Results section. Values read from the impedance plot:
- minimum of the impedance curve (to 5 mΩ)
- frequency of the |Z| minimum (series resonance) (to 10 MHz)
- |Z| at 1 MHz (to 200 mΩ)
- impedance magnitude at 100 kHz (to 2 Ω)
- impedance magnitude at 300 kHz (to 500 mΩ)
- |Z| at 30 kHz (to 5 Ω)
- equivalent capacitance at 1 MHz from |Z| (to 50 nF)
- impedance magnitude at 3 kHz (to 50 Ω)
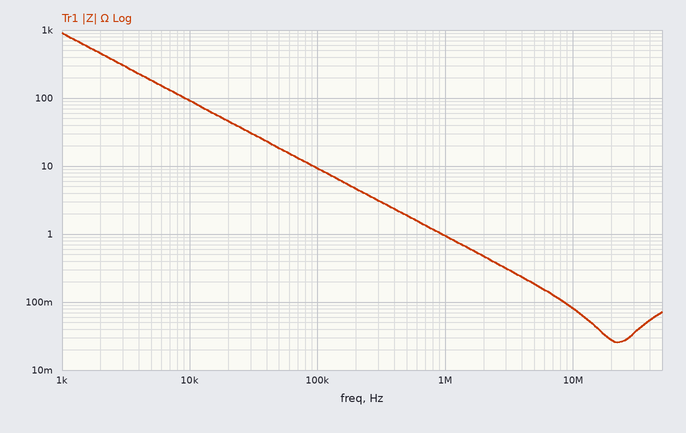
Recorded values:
25 mΩ
20 MHz
1.0 Ω
10 Ω
3.0 Ω
30 Ω
150 nF
300 Ω
